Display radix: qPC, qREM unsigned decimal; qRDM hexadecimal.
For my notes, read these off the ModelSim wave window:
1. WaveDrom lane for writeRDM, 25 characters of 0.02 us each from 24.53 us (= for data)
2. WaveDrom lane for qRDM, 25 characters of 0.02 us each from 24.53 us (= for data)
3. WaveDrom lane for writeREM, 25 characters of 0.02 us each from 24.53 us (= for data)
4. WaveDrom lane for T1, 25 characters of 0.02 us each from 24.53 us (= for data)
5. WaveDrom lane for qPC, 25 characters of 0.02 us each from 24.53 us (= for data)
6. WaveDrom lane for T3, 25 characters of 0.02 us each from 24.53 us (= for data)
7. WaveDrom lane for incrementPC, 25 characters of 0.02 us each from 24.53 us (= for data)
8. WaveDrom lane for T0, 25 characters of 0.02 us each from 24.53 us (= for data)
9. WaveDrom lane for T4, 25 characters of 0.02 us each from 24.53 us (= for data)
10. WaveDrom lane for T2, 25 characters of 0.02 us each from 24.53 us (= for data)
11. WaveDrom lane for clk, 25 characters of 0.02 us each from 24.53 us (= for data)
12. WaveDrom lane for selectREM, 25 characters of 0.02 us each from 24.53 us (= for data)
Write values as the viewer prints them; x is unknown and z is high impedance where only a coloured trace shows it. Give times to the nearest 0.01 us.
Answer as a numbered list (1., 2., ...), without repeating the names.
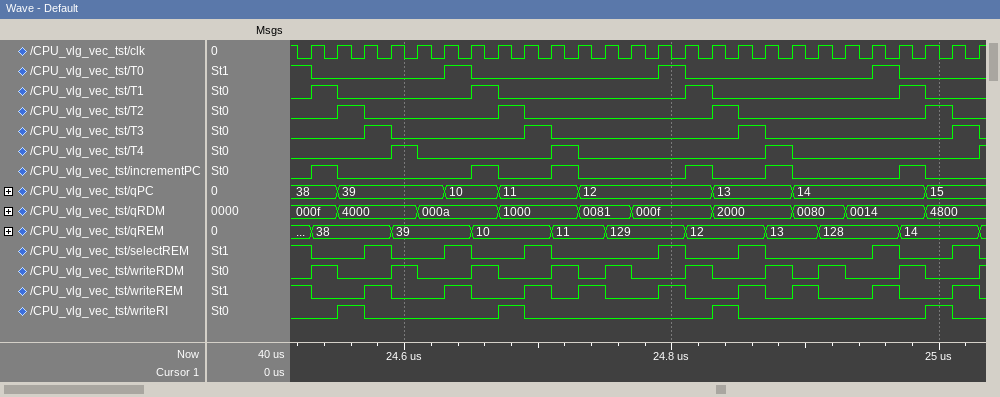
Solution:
1. {name: 'writeRDM', wave: '10.10.10.1010.10.1010.10.'}
2. {name: 'qRDM', wave: '==..=..=..=.=..=..=.=..=.', data: '000f 4000 000a 1000 0081 000f 2000 0080 0014 4800'}
3. {name: 'writeREM', wave: '0.10.10.1010.10.1010.10.1'}
4. {name: 'T1', wave: '10....10......10......10.'}
5. {name: 'qPC', wave: '==...=.=..=....=..=....=.', data: '38 39 10 11 12 13 14 15'}
6. {name: 'T3', wave: '0.10....10......10......1'}
7. {name: 'incrementPC', wave: '10....10.10...10.10...10.'}
8. {name: 'T0', wave: '0....10......10......10..'}
9. {name: 'T4', wave: '0..10....10......10......'}
10. {name: 'T2', wave: '010....10......10......10'}
11. {name: 'clk', wave: 'p........................'}
12. {name: 'selectREM', wave: '0.10.10.10...10.10...10.1'}
